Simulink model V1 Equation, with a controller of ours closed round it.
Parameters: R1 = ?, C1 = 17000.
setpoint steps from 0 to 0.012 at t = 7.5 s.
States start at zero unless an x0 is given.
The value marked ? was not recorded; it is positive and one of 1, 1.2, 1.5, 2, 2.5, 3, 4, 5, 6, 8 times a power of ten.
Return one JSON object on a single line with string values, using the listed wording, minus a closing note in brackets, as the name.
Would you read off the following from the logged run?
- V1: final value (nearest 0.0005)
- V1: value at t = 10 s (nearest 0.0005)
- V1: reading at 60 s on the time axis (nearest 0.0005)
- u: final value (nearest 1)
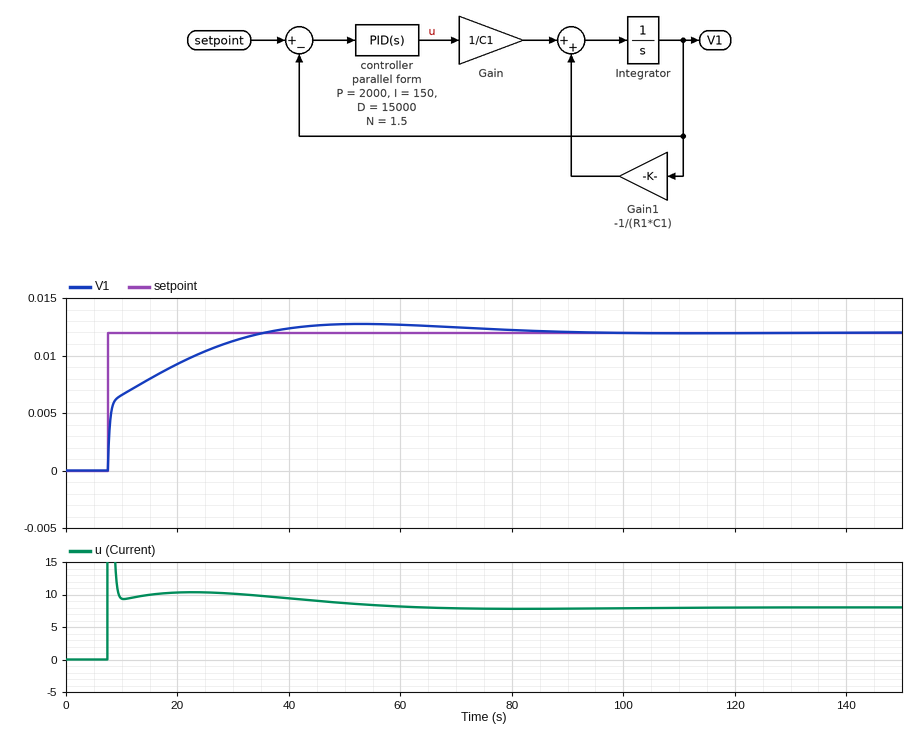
{"V1: final value": "0.0120", "V1: value at t = 10 s": "0.0065", "V1: reading at 60 s on the time axis": "0.0125", "u: final value": "8"}
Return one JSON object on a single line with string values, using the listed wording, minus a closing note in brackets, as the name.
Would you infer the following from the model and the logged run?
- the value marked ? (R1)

{"the value marked ?": "0.0015"}
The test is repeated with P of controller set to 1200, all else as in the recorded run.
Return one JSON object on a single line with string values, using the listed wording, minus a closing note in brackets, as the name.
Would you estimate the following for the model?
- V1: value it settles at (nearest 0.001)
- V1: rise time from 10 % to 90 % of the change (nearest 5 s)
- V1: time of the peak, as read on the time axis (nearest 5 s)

{"V1: value it settles at": "0.012", "V1: rise time from 10 % to 90 % of the change": "20 s", "V1: time of the peak, as read on the time axis": "55 s"}
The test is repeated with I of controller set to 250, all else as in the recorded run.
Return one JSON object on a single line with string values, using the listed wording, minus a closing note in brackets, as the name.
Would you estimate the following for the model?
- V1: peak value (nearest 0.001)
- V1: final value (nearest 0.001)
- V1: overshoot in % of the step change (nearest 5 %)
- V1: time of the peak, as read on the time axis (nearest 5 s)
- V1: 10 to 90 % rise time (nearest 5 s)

{"V1: peak value": "0.013", "V1: final value": "0.012", "V1: overshoot in % of the step change": "10 %", "V1: time of the peak, as read on the time axis": "40 s", "V1: 10 to 90 % rise time": "15 s"}
